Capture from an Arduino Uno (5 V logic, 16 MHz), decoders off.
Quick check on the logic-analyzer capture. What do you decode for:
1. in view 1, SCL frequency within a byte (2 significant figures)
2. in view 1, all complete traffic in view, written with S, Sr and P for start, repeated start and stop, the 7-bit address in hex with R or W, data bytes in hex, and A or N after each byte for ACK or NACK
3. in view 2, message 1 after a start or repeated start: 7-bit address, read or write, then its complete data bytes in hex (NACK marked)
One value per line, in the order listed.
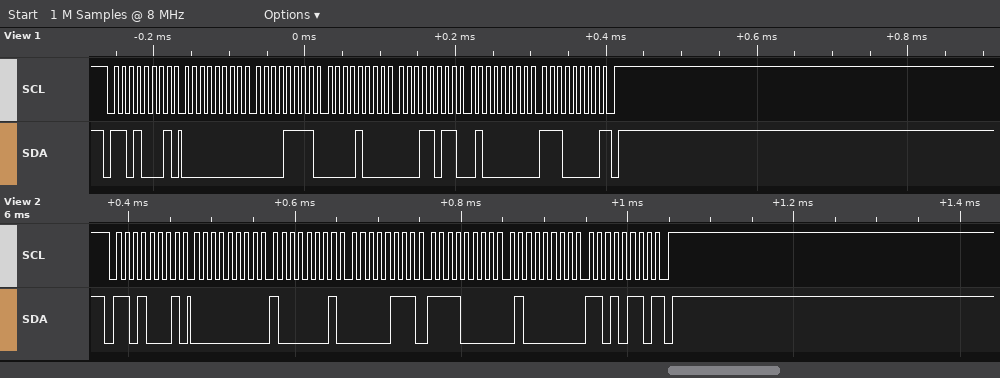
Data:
100 kHz
S 68R A 00 A 0F A 08 A 1B A 40 A E0 N P
0x68 read: 00 81 07 F0 40 D6 NACK
